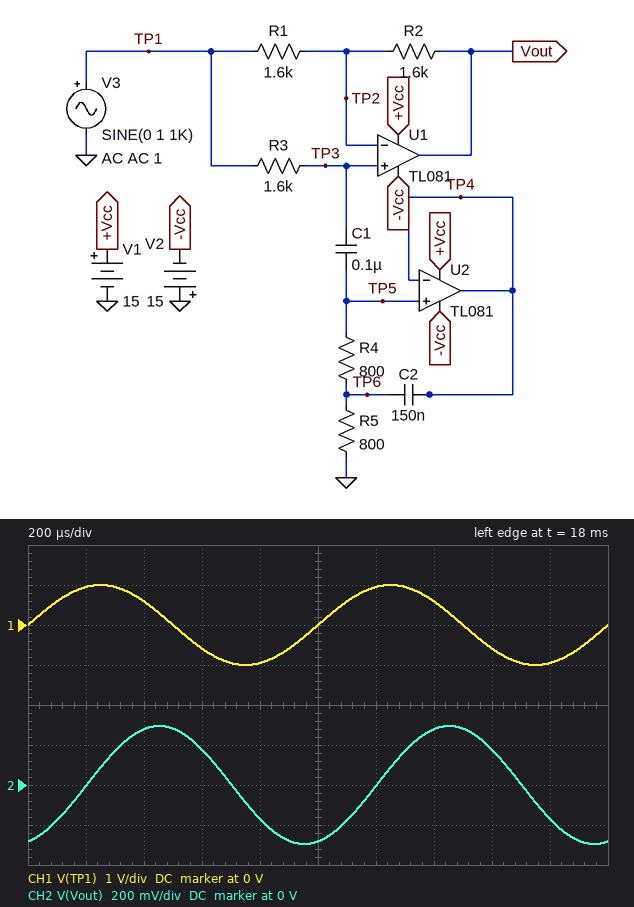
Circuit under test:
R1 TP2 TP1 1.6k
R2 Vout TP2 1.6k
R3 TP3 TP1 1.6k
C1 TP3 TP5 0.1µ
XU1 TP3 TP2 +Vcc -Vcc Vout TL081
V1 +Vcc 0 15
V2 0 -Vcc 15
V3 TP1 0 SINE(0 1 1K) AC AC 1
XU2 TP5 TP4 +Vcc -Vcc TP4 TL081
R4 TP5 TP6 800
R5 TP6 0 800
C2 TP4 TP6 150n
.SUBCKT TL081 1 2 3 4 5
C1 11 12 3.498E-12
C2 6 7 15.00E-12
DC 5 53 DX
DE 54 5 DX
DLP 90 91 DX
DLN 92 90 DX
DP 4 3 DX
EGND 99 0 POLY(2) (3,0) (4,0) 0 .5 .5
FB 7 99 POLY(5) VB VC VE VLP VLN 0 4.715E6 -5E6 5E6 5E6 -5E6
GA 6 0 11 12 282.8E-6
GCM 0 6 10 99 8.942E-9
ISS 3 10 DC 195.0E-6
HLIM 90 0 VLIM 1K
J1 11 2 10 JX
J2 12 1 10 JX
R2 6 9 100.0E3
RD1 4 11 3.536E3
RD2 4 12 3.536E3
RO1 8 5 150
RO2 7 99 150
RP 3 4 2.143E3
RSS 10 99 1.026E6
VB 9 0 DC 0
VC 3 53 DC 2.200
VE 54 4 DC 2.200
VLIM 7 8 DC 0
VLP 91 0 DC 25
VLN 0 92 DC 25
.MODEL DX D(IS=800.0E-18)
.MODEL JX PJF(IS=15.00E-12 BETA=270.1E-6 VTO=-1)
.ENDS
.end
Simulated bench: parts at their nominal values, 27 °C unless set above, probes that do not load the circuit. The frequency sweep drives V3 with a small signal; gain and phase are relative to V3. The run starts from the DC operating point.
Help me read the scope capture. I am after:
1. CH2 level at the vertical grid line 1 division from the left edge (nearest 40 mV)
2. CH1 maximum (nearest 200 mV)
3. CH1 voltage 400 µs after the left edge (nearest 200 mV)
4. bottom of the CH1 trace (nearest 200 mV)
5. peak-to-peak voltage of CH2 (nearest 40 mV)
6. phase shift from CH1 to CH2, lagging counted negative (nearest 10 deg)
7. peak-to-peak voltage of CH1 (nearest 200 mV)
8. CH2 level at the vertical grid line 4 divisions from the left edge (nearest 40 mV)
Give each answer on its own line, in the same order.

0 V
1.0 V
600 mV
-1.0 V
600 mV
-70 deg
2.0 V
-160 mV
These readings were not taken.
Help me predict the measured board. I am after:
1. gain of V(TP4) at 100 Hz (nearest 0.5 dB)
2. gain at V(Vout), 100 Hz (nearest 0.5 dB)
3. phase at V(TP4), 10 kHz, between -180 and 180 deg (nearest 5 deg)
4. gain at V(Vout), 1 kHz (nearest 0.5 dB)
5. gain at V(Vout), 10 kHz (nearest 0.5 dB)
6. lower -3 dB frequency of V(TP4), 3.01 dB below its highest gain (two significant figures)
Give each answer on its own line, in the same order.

-20.0 dB
0 dB
15 deg
-10.5 dB
-1.0 dB
3.1 kHz
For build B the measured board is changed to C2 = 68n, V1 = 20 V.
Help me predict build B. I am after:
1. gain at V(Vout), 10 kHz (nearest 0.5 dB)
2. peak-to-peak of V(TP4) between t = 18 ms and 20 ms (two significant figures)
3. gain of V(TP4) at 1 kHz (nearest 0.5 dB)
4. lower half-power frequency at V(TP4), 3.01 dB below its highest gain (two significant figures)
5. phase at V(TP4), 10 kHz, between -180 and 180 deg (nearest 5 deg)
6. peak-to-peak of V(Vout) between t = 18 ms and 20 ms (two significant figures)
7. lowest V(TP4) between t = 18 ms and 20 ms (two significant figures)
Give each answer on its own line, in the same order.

-4.0 dB
940 mV
-6.5 dB
7.5 kHz
20 deg
760 mV
-470 mV
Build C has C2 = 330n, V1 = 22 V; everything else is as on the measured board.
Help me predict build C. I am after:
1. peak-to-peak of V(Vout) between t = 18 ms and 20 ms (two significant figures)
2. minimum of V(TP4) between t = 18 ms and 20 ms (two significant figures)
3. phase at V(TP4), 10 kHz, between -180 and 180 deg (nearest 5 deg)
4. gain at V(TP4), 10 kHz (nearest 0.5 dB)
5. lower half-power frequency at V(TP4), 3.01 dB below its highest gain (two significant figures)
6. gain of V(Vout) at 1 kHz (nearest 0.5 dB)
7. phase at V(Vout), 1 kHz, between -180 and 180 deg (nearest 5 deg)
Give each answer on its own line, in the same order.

160 mV
-650 mV
5 deg
0 dB
1.2 kHz
-21.5 dB
-85 deg
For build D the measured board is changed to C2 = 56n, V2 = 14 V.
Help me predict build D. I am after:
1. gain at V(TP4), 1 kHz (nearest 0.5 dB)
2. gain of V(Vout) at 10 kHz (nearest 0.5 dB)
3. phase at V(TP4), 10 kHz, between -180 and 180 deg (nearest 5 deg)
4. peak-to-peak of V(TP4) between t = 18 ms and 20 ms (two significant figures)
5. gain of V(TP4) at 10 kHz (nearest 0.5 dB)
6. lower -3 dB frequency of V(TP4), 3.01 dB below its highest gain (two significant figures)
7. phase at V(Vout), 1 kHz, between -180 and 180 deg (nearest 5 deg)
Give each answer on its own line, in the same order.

-6.5 dB
-5.0 dB
20 deg
930 mV
-3.0 dB
9.2 kHz
-65 deg
